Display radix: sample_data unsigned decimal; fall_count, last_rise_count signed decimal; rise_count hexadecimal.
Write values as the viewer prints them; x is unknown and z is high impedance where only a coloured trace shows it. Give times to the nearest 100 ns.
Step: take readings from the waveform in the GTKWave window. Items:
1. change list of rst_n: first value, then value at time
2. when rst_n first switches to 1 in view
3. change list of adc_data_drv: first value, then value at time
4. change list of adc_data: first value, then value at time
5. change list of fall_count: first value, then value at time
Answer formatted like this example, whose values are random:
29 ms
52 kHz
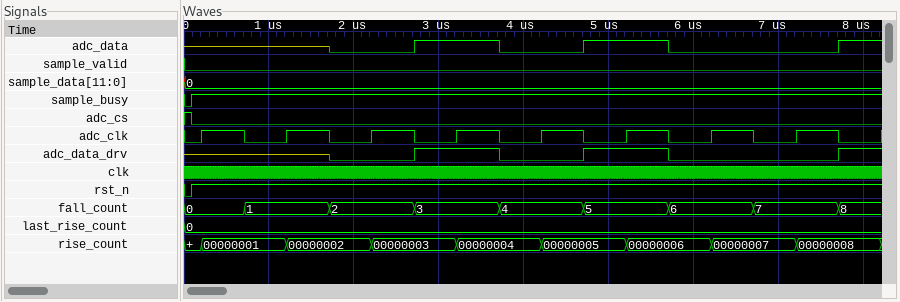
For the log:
0, 1 at 100 ns
100 ns
z, 0 at 1700 ns, 1 at 2700 ns, 0 at 3700 ns, 1 at 4700 ns, 0 at 5700 ns, 1 at 7700 ns
z, 0 at 1700 ns, 1 at 2700 ns, 0 at 3700 ns, 1 at 4700 ns, 0 at 5700 ns, 1 at 7700 ns
0, 1 at 700 ns, 2 at 1700 ns, 3 at 2700 ns, 4 at 3700 ns, 5 at 4700 ns, 6 at 5700 ns, 7 at 6700 ns, 8 at 7700 ns
